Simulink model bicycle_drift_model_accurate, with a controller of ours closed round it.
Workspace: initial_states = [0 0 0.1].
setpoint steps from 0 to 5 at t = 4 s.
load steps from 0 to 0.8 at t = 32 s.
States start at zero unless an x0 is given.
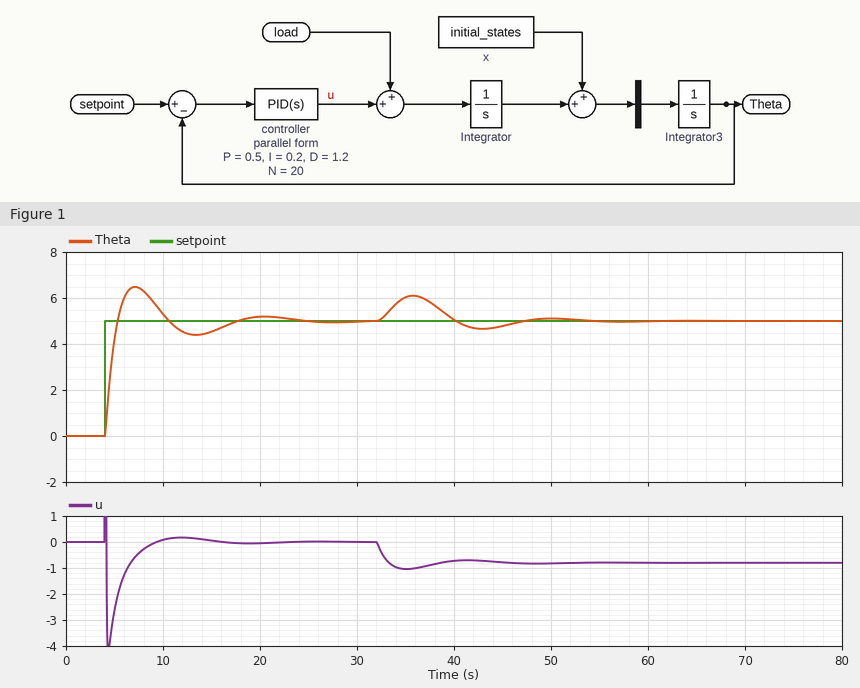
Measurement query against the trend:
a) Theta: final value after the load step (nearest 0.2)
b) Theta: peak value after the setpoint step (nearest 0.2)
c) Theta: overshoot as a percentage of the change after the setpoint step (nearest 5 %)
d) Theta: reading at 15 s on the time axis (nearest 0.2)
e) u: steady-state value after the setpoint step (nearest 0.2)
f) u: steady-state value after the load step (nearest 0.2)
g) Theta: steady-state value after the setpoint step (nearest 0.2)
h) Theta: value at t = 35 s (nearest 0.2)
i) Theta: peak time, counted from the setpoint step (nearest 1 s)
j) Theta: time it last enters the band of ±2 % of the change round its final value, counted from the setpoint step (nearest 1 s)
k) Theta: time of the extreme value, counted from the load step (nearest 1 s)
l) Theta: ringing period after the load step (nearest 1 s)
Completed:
5.0
6.4
30 %
4.6
0.0
-0.8
5.0
6.0
3 s
19 s
4 s
14 s
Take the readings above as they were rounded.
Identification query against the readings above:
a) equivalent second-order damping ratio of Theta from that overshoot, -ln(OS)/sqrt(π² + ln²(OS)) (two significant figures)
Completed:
0.36
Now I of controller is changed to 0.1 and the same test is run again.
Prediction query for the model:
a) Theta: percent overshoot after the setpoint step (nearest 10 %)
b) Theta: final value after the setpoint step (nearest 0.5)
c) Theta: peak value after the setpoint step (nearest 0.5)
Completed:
20 %
5.0
6.0
